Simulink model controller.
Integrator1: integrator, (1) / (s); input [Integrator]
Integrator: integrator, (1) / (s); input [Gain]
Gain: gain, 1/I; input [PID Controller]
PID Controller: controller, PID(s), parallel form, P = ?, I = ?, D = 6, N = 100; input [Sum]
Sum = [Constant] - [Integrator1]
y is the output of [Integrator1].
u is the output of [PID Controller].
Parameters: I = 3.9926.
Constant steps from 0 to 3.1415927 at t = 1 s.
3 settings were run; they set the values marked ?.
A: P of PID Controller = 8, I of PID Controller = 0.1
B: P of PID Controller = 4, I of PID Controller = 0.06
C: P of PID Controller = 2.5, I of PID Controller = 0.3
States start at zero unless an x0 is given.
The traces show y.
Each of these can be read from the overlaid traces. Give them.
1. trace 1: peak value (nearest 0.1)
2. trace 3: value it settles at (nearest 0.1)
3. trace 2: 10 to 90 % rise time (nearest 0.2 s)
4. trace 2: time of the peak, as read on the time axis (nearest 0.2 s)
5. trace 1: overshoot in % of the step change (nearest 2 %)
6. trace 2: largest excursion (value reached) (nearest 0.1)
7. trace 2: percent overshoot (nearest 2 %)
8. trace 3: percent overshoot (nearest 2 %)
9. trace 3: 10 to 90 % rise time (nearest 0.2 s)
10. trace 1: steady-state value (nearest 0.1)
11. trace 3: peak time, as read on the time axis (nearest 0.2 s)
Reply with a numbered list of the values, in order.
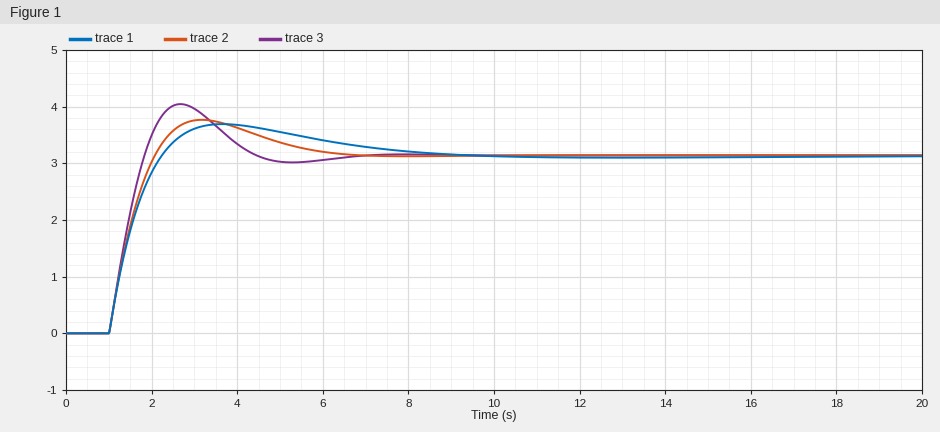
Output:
1. 3.7
2. 3.1
3. 0.8 s
4. 3.2 s
5. 18 %
6. 3.8
7. 20 %
8. 28 %
9. 0.6 s
10. 3.1
11. 2.6 s
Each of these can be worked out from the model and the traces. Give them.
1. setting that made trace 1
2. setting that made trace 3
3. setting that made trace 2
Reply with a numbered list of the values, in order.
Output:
1. C
2. A
3. B
